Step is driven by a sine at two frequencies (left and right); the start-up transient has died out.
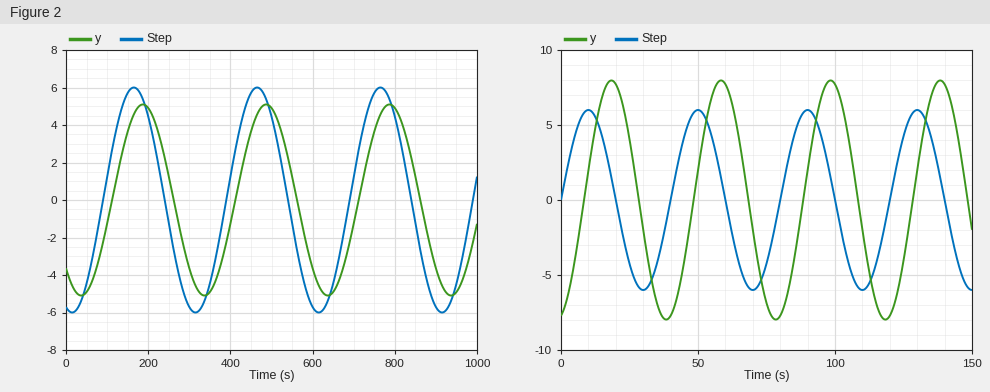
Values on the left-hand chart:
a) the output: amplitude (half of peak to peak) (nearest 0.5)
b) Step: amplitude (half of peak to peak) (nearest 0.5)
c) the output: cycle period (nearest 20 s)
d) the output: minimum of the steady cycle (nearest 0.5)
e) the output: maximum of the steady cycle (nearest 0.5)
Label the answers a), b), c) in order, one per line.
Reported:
a) 5.0
b) 6.0
c) 300 s
d) -5.0
e) 5.0
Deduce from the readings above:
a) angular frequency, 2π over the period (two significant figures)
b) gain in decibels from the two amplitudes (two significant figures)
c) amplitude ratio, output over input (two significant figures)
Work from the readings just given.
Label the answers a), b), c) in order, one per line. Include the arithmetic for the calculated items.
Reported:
a) 2π / 300 = 0.021 rad/s
b) 20 log10(5 / 6) = -1.6 dB
c) 5 / 6 = 0.83
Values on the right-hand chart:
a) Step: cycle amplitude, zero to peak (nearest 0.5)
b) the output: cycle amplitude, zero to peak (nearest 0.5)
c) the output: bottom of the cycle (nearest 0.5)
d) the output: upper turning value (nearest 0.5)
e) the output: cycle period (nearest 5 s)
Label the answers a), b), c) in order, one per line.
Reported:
a) 6.0
b) 8.0
c) -8.0
d) 8.0
e) 40 s
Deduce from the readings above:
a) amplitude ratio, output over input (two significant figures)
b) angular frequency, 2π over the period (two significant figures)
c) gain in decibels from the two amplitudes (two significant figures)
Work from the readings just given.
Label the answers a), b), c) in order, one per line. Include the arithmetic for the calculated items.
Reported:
a) 8 / 6 = 1.3
b) 2π / 40 = 0.16 rad/s
c) 20 log10(8 / 6) = 2.5 dB
